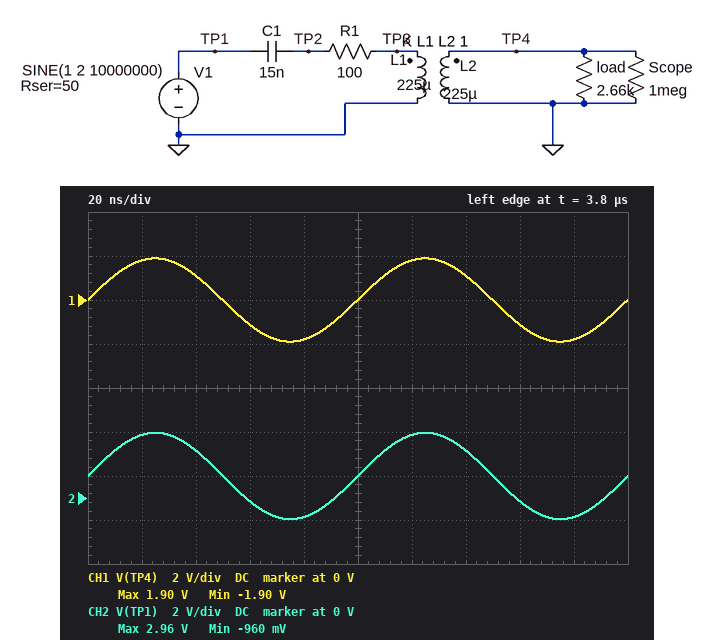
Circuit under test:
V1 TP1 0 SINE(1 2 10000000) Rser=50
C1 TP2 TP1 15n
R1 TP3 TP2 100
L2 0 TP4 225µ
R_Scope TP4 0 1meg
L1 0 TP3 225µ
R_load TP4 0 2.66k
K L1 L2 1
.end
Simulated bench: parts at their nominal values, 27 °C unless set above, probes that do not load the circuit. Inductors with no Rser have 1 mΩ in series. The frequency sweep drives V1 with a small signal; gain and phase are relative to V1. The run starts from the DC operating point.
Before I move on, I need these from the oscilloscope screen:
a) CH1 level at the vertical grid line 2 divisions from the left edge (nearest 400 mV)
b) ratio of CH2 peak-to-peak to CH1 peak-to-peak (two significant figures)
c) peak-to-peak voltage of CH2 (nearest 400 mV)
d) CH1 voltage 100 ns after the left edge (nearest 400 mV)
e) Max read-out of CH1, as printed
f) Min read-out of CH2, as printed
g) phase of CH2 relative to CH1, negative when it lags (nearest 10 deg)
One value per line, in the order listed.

1.2 V
1.0
4.0 V
0 V
1.90 V
-960 mV
0 deg
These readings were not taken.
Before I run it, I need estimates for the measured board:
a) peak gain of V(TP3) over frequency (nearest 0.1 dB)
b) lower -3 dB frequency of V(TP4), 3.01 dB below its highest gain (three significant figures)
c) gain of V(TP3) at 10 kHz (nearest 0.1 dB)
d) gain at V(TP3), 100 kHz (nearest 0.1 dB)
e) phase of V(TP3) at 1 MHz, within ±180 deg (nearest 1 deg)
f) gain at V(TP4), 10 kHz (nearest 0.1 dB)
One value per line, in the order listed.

-0.2 dB
76.7 kHz
-37.5 dB
-1.2 dB
6 deg
-37.5 dB
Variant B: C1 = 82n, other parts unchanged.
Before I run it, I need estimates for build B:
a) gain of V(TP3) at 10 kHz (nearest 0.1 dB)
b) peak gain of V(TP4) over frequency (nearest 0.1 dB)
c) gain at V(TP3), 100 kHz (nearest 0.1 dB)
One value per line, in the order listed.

-24.4 dB
-0.5 dB
-3.0 dB
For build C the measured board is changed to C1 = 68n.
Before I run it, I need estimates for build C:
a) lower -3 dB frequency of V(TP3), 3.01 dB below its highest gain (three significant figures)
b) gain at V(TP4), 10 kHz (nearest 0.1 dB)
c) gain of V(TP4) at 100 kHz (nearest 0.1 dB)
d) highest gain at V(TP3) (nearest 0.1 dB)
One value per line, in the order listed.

86.3 kHz
-25.5 dB
-2.9 dB
-0.5 dB
